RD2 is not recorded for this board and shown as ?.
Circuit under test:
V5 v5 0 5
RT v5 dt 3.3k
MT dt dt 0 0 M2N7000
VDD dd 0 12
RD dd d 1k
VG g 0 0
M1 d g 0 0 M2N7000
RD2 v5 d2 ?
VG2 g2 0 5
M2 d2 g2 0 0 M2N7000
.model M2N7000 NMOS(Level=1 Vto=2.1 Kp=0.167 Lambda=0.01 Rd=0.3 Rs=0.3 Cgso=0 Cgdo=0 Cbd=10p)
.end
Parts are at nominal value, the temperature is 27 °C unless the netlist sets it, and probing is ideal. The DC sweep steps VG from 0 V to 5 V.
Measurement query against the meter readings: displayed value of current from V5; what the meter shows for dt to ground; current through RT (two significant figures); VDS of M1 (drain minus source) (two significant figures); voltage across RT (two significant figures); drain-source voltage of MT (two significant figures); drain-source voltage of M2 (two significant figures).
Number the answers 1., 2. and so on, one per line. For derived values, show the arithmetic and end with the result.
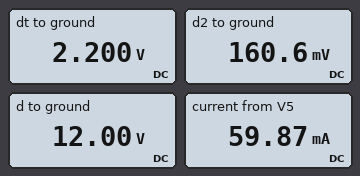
1. 59.87 mA
2. 2.200 V
3. (5 V - 2.2 V) / 3.3 kΩ = 850 µA
4. 12 V = 12 V
5. 5 V - 2.2 V = 2.8 V
6. 2.2 V = 2.2 V
7. 160.6 mV = 160 mV
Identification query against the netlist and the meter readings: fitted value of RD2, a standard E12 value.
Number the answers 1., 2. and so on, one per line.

1. 82 Ω
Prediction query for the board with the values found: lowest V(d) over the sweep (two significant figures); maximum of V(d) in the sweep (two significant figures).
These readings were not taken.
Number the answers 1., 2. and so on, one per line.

1. 32 mV
2. 12 V
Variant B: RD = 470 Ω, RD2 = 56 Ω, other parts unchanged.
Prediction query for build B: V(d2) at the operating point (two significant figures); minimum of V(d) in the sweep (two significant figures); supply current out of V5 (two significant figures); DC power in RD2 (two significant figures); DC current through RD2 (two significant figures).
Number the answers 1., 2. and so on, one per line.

1. 230 mV
2. 68 mV
3. 86 mA
4. 410 mW
5. 85 mA
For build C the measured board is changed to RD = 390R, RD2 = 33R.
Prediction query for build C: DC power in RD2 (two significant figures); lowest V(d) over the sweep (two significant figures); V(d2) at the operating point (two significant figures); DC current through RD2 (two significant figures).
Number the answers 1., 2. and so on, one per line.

1. 640 mW
2. 82 mV
3. 390 mV
4. 140 mA
